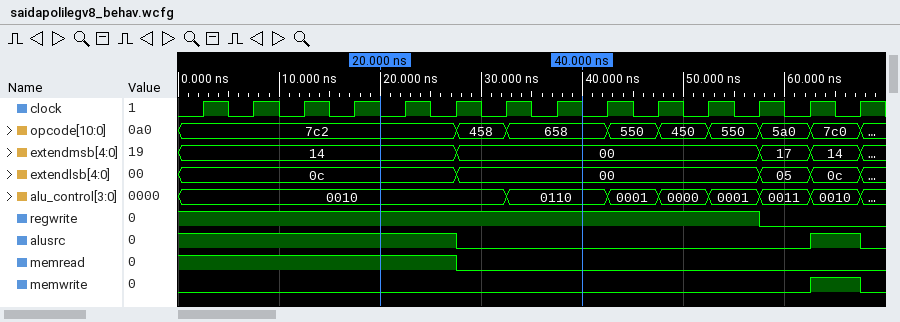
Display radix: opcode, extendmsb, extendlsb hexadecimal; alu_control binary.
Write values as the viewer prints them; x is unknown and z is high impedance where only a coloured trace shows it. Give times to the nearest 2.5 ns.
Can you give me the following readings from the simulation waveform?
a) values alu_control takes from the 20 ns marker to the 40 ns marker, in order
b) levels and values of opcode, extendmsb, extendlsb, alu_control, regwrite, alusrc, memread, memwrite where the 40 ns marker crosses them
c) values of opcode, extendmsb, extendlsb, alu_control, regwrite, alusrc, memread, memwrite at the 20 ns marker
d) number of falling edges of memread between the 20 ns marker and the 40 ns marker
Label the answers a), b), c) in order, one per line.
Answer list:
a) 0010, 0110
b) opcode=658, extendmsb=00, extendlsb=00, alu_control=0110, regwrite=1, alusrc=0, memread=0, memwrite=0
c) opcode=7c2, extendmsb=14, extendlsb=0c, alu_control=0010, regwrite=1, alusrc=1, memread=1, memwrite=0
d) 1
